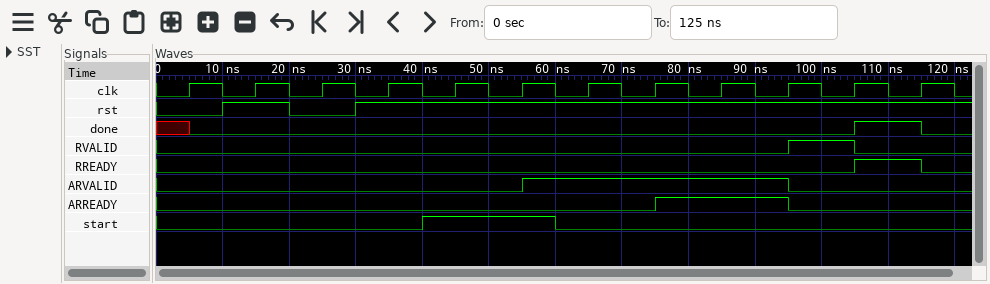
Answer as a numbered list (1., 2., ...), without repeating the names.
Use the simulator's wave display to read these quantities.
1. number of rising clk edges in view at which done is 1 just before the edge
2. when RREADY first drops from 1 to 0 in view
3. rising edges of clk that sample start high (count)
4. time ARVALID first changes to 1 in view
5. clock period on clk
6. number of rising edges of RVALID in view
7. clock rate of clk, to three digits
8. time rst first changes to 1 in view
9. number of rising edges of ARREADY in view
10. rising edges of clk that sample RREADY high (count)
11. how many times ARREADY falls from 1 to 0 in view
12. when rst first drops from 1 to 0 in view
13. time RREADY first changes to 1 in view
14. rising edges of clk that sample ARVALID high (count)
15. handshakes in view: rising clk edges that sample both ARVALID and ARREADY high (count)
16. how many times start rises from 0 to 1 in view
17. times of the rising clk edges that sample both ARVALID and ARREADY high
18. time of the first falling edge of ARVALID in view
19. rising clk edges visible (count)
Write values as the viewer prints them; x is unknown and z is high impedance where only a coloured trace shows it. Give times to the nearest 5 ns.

1. 1
2. 115 ns
3. 2
4. 55 ns
5. 10 ns
6. 1
7. 100 MHz
8. 10 ns
9. 1
10. 1
11. 1
12. 20 ns
13. 105 ns
14. 4
15. 2
16. 1
17. 85 ns, 95 ns
18. 95 ns
19. 12
